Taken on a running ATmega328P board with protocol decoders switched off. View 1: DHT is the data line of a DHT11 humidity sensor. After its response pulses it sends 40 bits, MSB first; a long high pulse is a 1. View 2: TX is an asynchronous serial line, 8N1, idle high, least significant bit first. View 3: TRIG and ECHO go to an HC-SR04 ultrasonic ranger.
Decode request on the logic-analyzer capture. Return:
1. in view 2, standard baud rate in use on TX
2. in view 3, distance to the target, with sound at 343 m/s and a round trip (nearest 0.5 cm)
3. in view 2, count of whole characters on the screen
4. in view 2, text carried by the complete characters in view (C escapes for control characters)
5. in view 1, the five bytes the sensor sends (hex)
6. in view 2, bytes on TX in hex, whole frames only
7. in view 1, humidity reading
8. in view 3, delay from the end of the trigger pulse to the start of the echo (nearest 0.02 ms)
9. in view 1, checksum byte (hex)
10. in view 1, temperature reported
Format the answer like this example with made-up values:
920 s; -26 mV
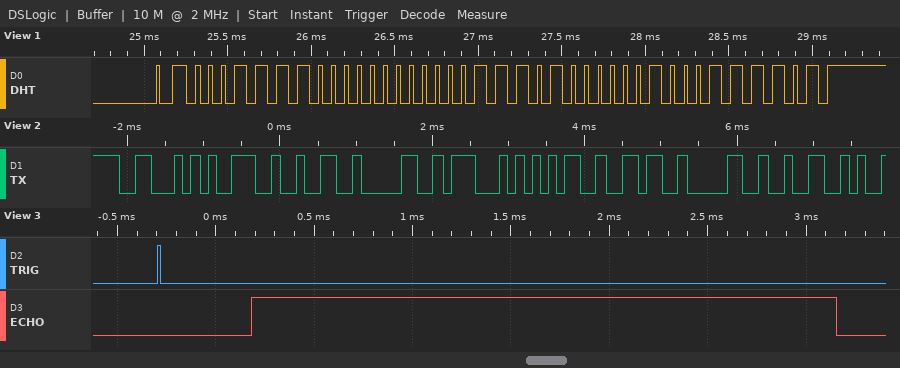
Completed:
9600 baud; 51 cm; 9; "F920G5602"; 1E 00 1D 02 3D; 0x46 0x39 0x32 0x30 0x47 0x35 0x36 0x30 0x32; 30 %; 0.46 ms; 0x3D; 29.2 °C
